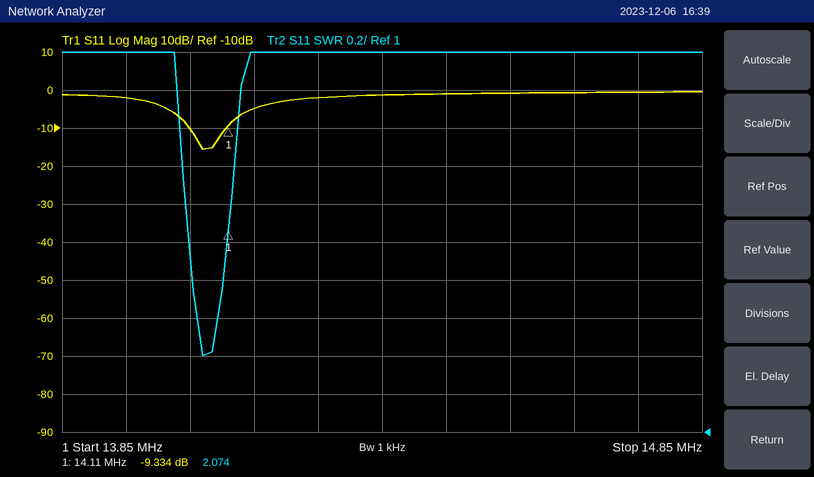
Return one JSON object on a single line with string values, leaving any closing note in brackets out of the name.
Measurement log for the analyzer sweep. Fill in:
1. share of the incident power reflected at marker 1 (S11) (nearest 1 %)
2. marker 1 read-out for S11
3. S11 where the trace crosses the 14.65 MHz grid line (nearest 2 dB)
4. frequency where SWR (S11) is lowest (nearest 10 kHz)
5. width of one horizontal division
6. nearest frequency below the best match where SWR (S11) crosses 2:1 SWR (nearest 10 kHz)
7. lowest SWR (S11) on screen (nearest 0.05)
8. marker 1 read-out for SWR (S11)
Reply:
{"share of the incident power reflected at marker 1 (S11)": "12 %", "marker 1 read-out for S11": "-9.334 dB", "S11 where the trace crosses the 14.65 MHz grid line": "0 dB", "frequency where SWR (S11) is lowest": "14.07 MHz", "width of one horizontal division": "100 kHz", "nearest frequency below the best match where SWR (S11) crosses 2:1 SWR": "14.05 MHz", "lowest SWR (S11) on screen": "1.40", "marker 1 read-out for SWR": "2.074"}
